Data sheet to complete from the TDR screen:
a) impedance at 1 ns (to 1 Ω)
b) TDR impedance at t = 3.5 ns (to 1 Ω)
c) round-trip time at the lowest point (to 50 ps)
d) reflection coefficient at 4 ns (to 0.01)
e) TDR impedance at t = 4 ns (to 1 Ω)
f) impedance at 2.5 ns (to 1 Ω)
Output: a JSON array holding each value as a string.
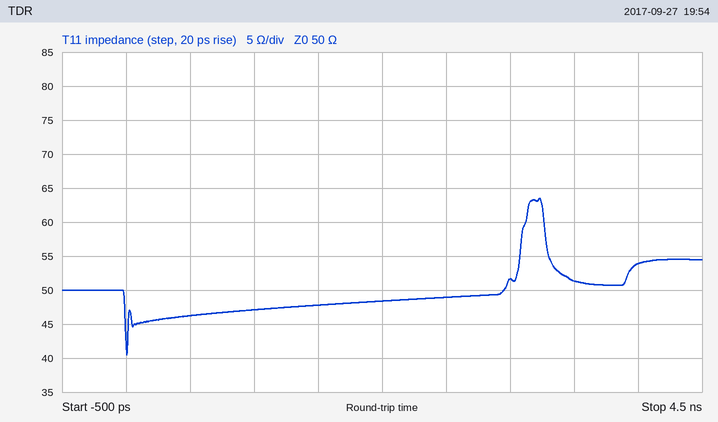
["47 Ω", "51 Ω", "0 ps", "+0.04", "54 Ω", "49 Ω"]
